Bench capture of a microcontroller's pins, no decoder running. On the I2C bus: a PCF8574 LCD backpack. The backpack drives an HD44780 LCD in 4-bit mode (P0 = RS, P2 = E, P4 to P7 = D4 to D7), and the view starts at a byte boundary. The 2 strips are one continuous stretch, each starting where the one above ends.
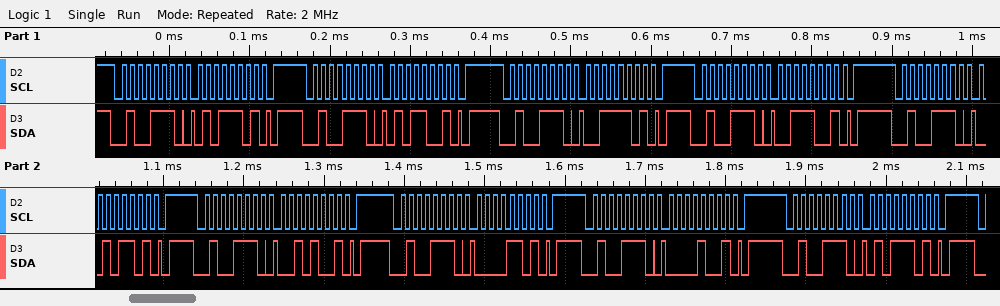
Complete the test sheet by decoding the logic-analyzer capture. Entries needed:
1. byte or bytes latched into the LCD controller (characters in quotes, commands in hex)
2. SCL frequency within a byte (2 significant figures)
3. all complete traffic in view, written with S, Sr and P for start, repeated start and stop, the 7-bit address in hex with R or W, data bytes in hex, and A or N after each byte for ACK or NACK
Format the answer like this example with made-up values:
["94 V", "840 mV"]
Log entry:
["'S' ' '", "100 kHz", "S 27W A 5D A P S 27W A 59 A P S 27W A 3D A P S 27W A 39 A P S 27W A 2D A P S 27W A 29 A P S 27W A 0D A P S 27W A 09 A P S 27W A 5D A P"]
